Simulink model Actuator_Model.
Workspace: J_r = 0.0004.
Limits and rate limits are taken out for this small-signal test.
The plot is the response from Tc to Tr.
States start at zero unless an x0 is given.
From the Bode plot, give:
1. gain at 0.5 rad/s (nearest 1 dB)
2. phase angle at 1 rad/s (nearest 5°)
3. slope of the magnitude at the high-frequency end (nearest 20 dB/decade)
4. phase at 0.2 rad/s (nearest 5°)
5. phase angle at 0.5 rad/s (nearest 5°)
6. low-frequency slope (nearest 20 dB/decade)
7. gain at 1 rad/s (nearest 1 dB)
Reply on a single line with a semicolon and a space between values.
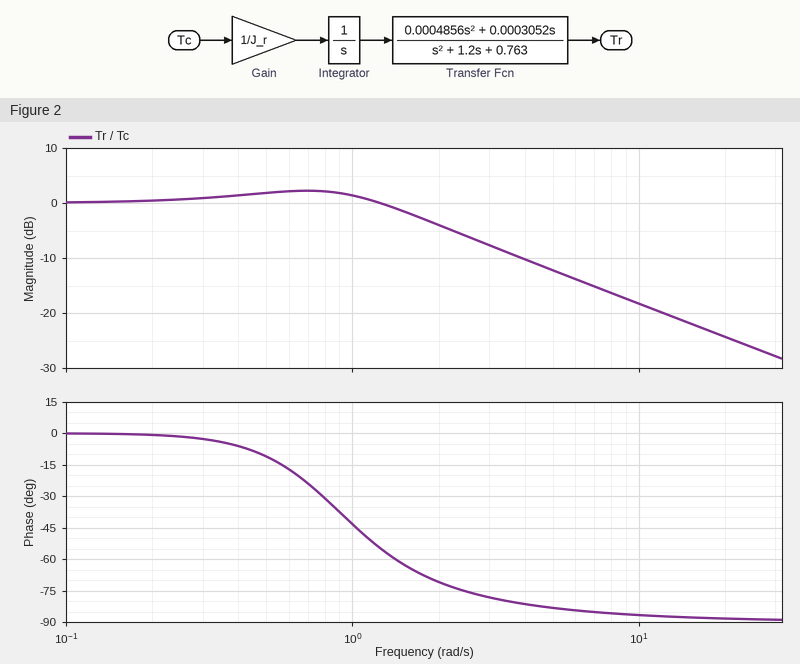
2 dB; -45°; -20 dB/decade; 0°; -10°; 0 dB/decade; 1 dB
